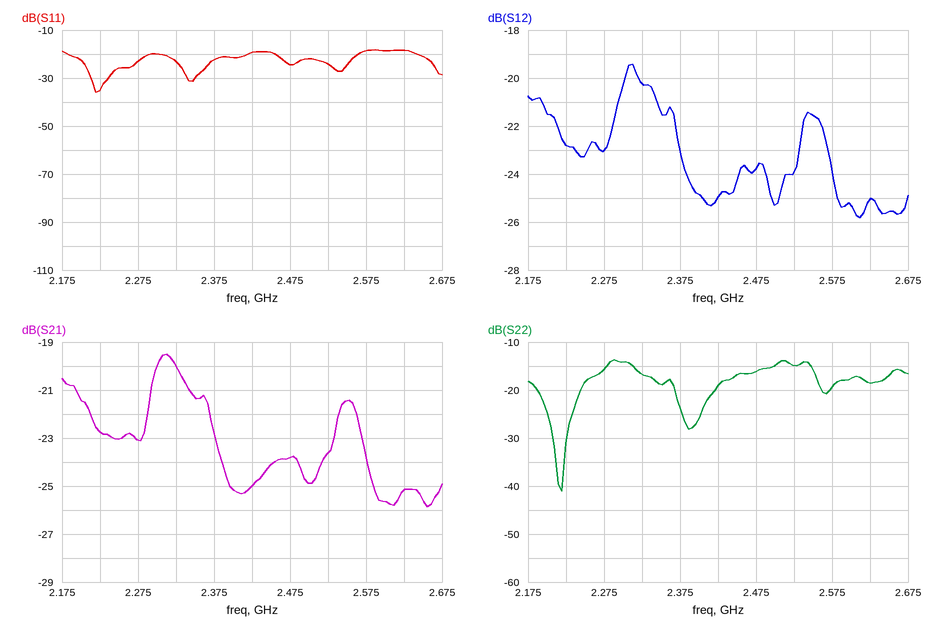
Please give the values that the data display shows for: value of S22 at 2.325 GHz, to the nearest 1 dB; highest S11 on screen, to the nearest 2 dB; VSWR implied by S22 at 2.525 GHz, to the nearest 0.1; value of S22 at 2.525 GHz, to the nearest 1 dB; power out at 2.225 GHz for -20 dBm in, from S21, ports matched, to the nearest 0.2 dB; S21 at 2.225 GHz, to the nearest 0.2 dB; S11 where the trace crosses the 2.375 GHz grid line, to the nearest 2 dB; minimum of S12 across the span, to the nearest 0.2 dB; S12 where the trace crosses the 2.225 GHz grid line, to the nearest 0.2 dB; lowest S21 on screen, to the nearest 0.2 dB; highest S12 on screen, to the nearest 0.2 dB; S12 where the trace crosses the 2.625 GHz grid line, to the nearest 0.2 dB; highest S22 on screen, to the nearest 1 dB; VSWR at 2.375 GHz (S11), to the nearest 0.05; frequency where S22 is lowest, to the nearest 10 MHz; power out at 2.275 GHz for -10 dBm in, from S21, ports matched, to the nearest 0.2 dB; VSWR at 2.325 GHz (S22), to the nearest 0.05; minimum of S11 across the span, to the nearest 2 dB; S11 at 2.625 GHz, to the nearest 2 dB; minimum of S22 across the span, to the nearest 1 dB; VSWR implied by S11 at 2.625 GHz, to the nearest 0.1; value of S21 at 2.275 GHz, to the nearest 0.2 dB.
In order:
-17 dB
-18 dB
1.4
-15 dB
-42.8 dBm
-22.8 dB
-22 dB
-25.8 dB
-22.8 dB
-25.8 dB
-19.4 dB
-25.0 dB
-14 dB
1.15
2.22 GHz
-33.0 dBm
1.35
-36 dB
-18 dB
-41 dB
1.3
-23.0 dB
